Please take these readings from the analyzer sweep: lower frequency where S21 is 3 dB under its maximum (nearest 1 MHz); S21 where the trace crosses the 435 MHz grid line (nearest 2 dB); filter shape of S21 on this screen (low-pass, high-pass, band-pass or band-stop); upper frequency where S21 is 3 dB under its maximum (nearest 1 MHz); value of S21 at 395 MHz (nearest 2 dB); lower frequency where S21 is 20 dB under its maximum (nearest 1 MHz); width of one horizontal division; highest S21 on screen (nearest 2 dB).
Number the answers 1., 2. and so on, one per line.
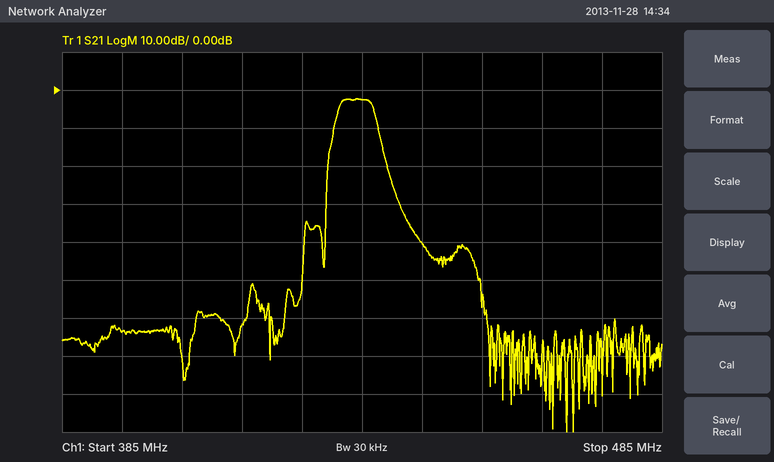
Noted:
1. 431 MHz
2. -2 dB
3. band-pass
4. 437 MHz
5. -64 dB
6. 429 MHz
7. 10 MHz
8. -2 dB
